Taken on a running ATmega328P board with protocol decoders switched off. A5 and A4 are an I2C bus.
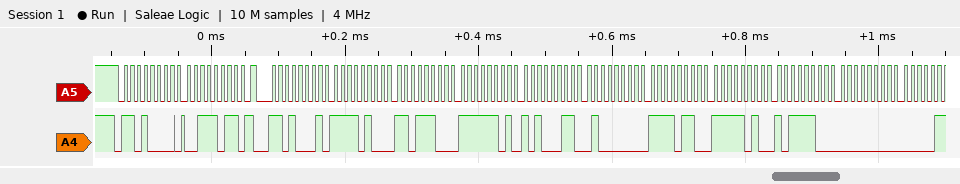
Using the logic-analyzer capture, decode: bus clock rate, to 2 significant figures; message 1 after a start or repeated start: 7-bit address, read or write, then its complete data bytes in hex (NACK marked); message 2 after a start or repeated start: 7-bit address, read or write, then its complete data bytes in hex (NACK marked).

100 kHz
0x68 write: 3B
0x68 read: F4 DC FD A3 40 F6 FA BC 00
